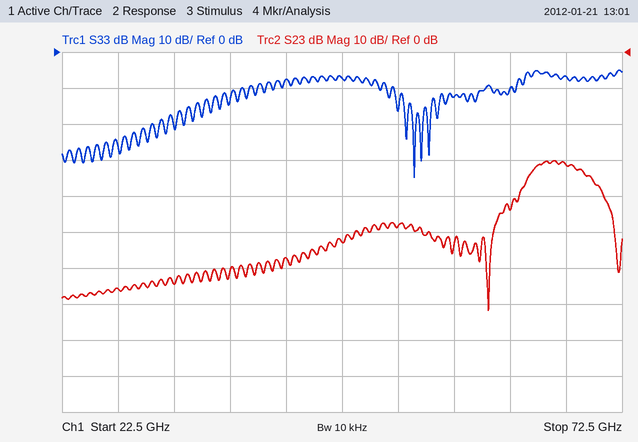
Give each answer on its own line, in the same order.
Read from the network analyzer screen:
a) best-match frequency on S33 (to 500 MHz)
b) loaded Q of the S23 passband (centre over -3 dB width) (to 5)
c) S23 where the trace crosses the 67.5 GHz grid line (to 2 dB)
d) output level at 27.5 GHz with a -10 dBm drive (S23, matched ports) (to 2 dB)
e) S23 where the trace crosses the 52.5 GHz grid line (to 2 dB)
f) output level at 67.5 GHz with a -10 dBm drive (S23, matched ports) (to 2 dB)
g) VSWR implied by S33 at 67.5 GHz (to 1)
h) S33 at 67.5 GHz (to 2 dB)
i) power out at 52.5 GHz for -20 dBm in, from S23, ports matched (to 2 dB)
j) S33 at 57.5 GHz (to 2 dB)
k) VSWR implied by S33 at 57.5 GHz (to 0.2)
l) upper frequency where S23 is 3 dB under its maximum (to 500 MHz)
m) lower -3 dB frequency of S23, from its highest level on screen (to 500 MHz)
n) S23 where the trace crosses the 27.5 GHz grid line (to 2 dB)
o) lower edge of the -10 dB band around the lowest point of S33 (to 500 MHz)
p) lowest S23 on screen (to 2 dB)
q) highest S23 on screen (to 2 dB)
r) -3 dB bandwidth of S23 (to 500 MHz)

54.0 GHz
15
-32 dB
-76 dBm
-48 dB
-42 dBm
3
-6 dB
-68 dBm
-12 dB
1.6
69.0 GHz
64.5 GHz
-66 dB
52.0 GHz
-72 dB
-30 dB
4.5 GHz
